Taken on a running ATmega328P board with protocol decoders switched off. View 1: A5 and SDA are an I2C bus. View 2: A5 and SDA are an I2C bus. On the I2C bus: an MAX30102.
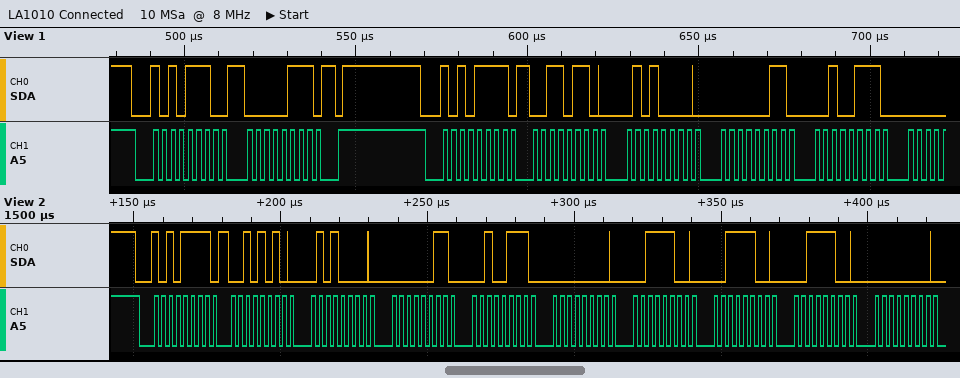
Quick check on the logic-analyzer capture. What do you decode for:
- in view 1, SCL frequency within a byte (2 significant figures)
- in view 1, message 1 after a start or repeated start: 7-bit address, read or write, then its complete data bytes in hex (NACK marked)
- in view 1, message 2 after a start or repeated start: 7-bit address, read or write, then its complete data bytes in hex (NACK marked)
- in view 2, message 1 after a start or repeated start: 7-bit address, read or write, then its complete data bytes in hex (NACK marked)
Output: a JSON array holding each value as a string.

["400 kHz", "0x57 write: 07", "0x57 read: 36 50 03 27", "0x57 read: 2A 50 03 27 00 3C 3C 3C 00"]
